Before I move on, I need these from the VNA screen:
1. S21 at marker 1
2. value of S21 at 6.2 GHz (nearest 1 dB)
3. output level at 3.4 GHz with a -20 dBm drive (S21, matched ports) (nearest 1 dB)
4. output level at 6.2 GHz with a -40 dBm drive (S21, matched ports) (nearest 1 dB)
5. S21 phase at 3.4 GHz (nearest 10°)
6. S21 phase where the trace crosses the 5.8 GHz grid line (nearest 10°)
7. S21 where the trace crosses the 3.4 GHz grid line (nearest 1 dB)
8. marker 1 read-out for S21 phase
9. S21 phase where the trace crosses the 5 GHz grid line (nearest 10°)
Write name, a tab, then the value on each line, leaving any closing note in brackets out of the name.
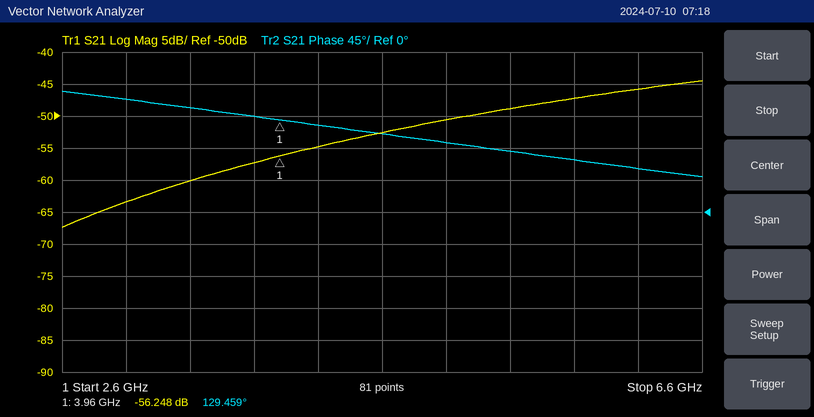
S21 at marker 1	-56.248 dB
value of S21 at 6.2 GHz	-46 dB
output level at 3.4 GHz with a -20 dBm drive (S21, matched ports)	-80 dBm
output level at 6.2 GHz with a -40 dBm drive (S21, matched ports)	-86 dBm
S21 phase at 3.4 GHz	150°
S21 phase where the trace crosses the 5.8 GHz grid line	70°
S21 where the trace crosses the 3.4 GHz grid line	-60 dB
marker 1 read-out for S21 phase	129.459°
S21 phase where the trace crosses the 5 GHz grid line	100°
